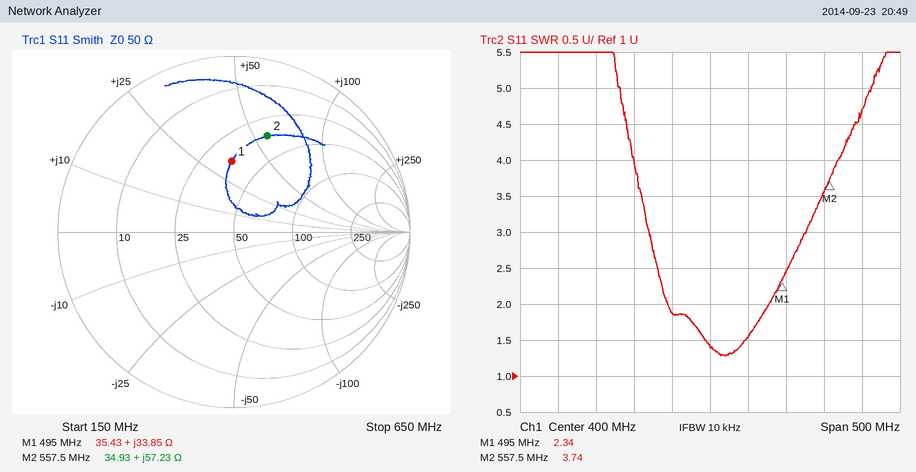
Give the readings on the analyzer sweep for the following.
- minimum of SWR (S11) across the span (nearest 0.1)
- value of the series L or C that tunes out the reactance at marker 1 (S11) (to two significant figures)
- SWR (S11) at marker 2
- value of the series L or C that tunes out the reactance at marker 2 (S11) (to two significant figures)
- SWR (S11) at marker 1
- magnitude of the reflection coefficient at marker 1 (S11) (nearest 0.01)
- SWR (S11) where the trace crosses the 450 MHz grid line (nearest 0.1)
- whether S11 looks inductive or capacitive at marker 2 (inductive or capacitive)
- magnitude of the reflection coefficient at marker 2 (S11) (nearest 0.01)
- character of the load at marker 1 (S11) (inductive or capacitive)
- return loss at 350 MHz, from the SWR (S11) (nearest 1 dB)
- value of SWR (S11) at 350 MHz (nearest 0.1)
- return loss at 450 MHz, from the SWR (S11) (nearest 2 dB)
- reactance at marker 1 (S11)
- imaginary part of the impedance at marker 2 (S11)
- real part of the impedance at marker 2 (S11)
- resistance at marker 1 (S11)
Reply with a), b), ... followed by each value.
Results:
a) 1.3
b) 9.5 pF
c) 3.74
d) 5.0 pF
e) 2.34
f) 0.40
g) 1.5
h) inductive
i) 0.58
j) inductive
k) 10 dB
l) 1.9
m) 14 dB
n) +33.85 Ω
o) +57.23 Ω
p) 34.93 Ω
q) 35.43 Ω
